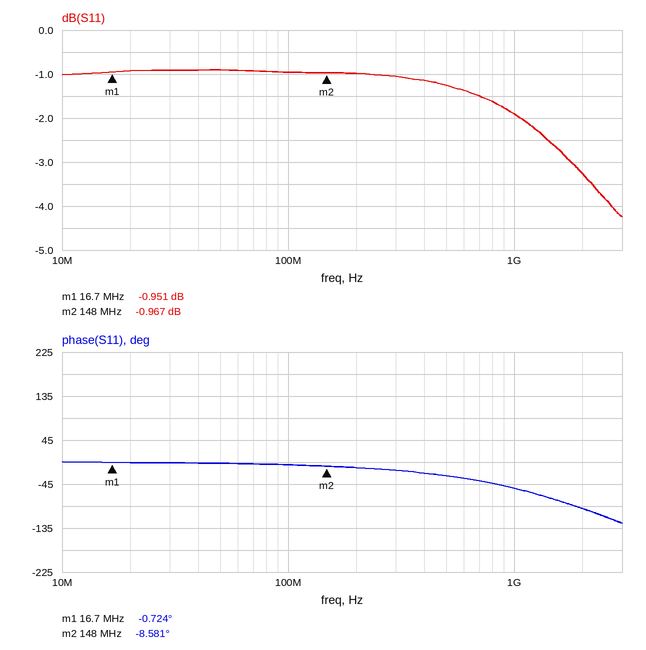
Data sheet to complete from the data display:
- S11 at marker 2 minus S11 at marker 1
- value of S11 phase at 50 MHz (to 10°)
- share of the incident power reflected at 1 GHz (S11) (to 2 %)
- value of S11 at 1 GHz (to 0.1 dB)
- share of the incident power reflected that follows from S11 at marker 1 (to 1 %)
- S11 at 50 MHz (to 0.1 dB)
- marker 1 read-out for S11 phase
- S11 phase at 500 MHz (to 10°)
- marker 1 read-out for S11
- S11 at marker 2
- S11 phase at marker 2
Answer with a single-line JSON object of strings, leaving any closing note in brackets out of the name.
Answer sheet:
{"S11 at marker 2 minus S11 at marker 1": "-0.016 dB", "value of S11 phase at 50 MHz": "0°", "share of the incident power reflected at 1 GHz (S11)": "64 %", "value of S11 at 1 GHz": "-1.9 dB", "share of the incident power reflected that follows from S11 at marker 1": "80 %", "S11 at 50 MHz": "-0.9 dB", "marker 1 read-out for S11 phase": "-0.724°", "S11 phase at 500 MHz": "-30°", "marker 1 read-out for S11": "-0.951 dB", "S11 at marker 2": "-0.967 dB", "S11 phase at marker 2": "-8.581°"}
